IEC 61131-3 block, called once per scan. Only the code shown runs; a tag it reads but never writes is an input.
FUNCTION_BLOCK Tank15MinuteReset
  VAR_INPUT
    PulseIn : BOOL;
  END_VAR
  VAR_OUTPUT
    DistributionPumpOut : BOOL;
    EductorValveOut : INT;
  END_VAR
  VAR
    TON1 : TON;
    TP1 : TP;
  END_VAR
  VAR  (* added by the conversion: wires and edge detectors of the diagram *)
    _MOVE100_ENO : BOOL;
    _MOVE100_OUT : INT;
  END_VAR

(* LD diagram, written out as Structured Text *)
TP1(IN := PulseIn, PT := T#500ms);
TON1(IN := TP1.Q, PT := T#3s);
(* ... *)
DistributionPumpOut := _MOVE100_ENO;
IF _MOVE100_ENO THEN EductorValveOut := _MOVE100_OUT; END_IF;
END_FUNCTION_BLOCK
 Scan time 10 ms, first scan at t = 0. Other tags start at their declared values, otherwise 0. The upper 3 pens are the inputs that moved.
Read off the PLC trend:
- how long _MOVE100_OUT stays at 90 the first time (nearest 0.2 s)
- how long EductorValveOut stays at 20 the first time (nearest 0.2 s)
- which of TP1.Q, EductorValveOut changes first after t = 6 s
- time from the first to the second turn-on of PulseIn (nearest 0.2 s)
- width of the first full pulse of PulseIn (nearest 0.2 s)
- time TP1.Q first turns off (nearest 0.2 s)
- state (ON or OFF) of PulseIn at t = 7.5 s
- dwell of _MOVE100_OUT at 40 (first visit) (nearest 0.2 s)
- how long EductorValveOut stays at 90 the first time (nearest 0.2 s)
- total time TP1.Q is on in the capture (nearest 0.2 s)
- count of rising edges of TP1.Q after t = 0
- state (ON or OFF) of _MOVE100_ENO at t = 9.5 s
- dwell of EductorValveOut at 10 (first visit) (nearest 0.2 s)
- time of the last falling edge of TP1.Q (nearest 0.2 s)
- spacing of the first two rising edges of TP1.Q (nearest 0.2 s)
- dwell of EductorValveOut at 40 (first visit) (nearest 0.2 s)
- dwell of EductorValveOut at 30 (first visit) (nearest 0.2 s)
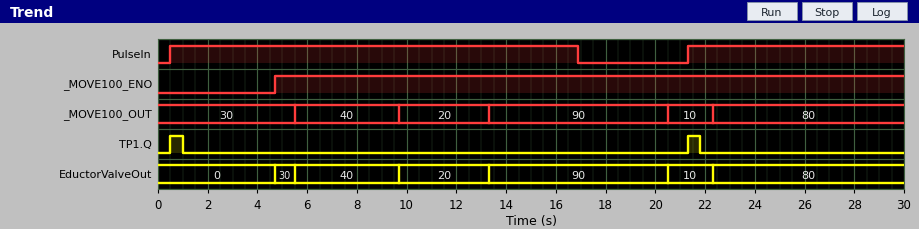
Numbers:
7.2 s
3.6 s
EductorValveOut
20.8 s
16.4 s
1.0 s
ON
4.2 s
7.2 s
1.0 s
2
ON
1.8 s
21.8 s
20.8 s
4.2 s
0.8 s
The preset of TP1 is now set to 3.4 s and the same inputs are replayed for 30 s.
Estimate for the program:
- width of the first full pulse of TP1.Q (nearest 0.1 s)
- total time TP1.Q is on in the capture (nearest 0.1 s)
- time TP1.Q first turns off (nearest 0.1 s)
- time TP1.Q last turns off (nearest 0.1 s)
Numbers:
3.4 s
6.8 s
3.9 s
24.7 s
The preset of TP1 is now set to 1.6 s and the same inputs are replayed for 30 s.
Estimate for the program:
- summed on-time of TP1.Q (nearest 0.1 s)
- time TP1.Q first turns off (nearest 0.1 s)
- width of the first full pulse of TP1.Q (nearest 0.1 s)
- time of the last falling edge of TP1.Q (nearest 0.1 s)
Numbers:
3.2 s
2.1 s
1.6 s
22.9 s
